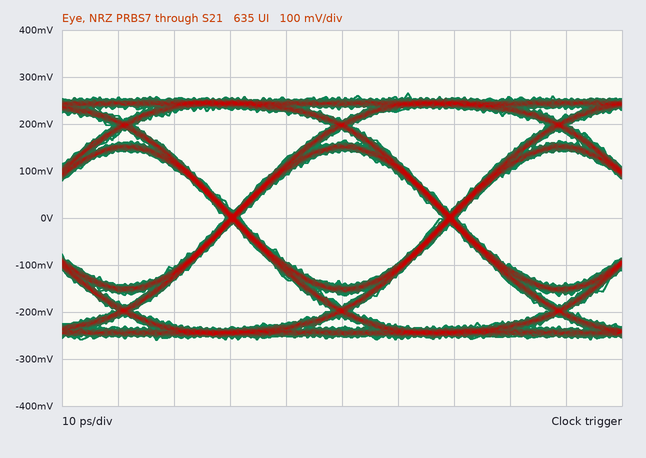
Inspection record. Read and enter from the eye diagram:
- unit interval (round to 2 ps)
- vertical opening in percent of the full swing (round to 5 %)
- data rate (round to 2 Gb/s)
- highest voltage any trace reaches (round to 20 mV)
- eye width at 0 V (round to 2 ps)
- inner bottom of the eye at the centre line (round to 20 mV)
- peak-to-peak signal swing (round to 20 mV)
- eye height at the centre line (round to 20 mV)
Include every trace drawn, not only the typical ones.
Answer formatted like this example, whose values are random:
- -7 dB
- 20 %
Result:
- 38 ps
- 55 %
- 26 Gb/s
- 260 mV
- 36 ps
- -140 mV
- 520 mV
- 280 mV
